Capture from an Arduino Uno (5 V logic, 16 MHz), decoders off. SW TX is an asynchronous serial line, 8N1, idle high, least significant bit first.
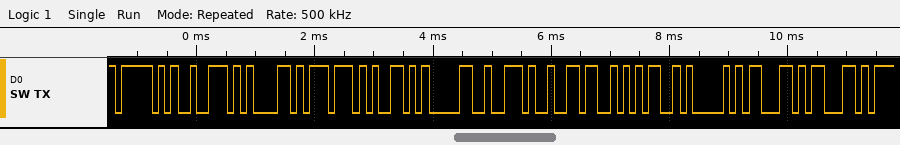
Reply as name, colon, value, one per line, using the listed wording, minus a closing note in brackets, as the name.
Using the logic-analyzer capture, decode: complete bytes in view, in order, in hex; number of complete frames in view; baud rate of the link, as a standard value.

complete bytes in view, in order, in hex: 0x5F 0x72 0x61 0x77 0x59 0x30 0x2E 0x36 0x35 0x41 0x63 0x63
number of complete frames in view: 12
baud rate of the link, as a standard value: 9600 baud
